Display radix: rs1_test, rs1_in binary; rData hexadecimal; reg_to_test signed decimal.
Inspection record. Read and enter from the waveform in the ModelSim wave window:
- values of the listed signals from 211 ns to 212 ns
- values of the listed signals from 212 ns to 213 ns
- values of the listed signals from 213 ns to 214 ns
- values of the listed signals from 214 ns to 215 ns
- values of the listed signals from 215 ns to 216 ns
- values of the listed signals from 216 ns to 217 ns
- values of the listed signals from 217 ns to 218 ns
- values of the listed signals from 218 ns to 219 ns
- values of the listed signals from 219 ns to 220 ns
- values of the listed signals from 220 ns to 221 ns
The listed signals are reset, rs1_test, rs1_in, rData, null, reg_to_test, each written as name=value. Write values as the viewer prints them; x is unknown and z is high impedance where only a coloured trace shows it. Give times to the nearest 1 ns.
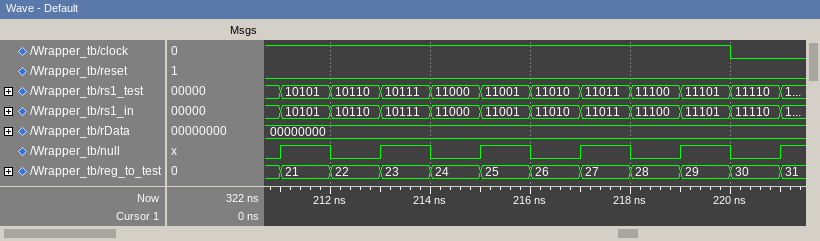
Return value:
reset=0, rs1_test=10101, rs1_in=10101, rData=00000000, null=1, reg_to_test=21
reset=0, rs1_test=10110, rs1_in=10110, rData=00000000, null=0, reg_to_test=22
reset=0, rs1_test=10111, rs1_in=10111, rData=00000000, null=1, reg_to_test=23
reset=0, rs1_test=11000, rs1_in=11000, rData=00000000, null=0, reg_to_test=24
reset=0, rs1_test=11001, rs1_in=11001, rData=00000000, null=1, reg_to_test=25
reset=0, rs1_test=11010, rs1_in=11010, rData=00000000, null=0, reg_to_test=26
reset=0, rs1_test=11011, rs1_in=11011, rData=00000000, null=1, reg_to_test=27
reset=0, rs1_test=11100, rs1_in=11100, rData=00000000, null=0, reg_to_test=28
reset=0, rs1_test=11101, rs1_in=11101, rData=00000000, null=1, reg_to_test=29
reset=0, rs1_test=11110, rs1_in=11110, rData=00000000, null=0, reg_to_test=30
